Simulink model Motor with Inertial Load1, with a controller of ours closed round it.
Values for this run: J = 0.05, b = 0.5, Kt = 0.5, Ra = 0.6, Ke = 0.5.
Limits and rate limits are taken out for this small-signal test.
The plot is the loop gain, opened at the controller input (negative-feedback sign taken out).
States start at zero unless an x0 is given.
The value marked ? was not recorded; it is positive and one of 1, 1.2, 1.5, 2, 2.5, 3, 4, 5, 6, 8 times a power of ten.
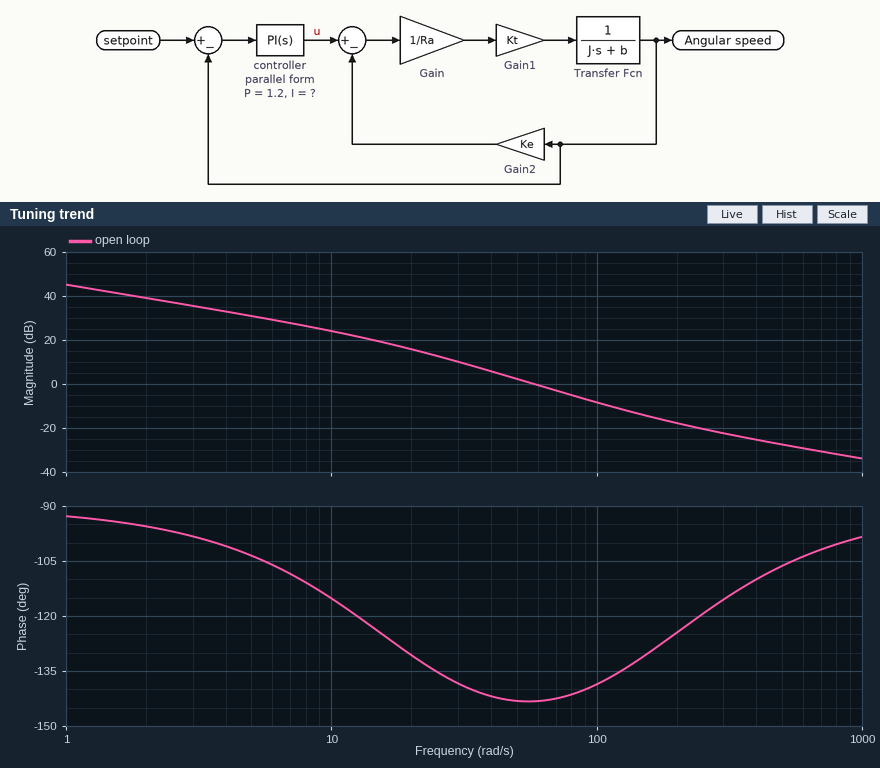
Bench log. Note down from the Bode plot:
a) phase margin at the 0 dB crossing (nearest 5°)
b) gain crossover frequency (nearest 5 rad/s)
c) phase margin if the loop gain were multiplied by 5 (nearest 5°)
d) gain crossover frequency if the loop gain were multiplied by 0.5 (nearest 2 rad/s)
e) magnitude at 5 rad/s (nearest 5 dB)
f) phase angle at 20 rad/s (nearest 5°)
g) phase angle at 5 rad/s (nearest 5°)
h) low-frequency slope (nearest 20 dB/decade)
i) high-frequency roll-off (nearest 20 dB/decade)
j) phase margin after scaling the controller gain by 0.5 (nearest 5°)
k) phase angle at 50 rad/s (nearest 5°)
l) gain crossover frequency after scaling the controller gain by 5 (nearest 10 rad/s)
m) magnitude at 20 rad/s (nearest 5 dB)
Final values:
35°
60 rad/s
50°
40 rad/s
30 dB
-130°
-105°
-20 dB/decade
-20 dB/decade
40°
-145°
150 rad/s
15 dB
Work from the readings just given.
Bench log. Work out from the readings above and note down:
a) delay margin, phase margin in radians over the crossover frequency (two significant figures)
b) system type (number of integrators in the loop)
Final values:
0.010 s
1
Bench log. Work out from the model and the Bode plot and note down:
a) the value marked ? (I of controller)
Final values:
200
